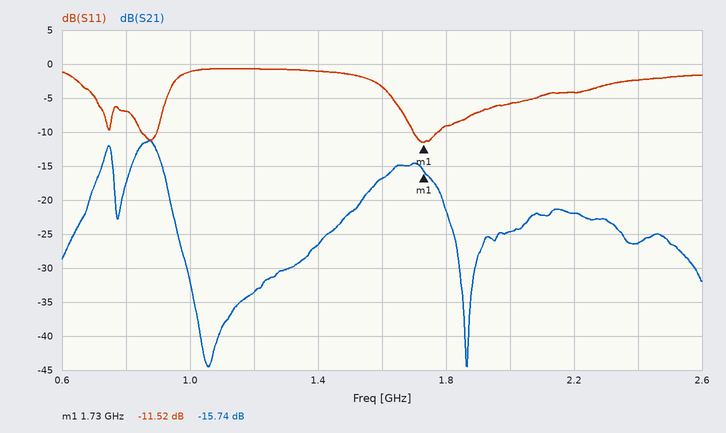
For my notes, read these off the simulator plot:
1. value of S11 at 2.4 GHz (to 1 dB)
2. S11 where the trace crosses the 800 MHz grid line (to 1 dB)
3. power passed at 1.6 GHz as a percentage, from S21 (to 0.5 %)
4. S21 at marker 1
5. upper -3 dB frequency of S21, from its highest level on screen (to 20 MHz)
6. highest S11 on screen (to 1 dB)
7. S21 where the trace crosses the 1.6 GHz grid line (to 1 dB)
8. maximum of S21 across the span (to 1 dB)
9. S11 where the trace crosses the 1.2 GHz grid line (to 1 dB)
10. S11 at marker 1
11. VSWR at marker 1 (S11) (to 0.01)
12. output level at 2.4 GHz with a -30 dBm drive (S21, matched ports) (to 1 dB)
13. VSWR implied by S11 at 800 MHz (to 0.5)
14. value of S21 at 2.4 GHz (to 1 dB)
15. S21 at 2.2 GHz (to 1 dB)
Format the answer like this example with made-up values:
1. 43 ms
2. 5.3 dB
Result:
1. -2 dB
2. -7 dB
3. 2.0 %
4. -15.74 dB
5. 900 MHz
6. -1 dB
7. -17 dB
8. -11 dB
9. -1 dB
10. -11.52 dB
11. 1.72
12. -56 dBm
13. 2.5
14. -26 dB
15. -22 dB
